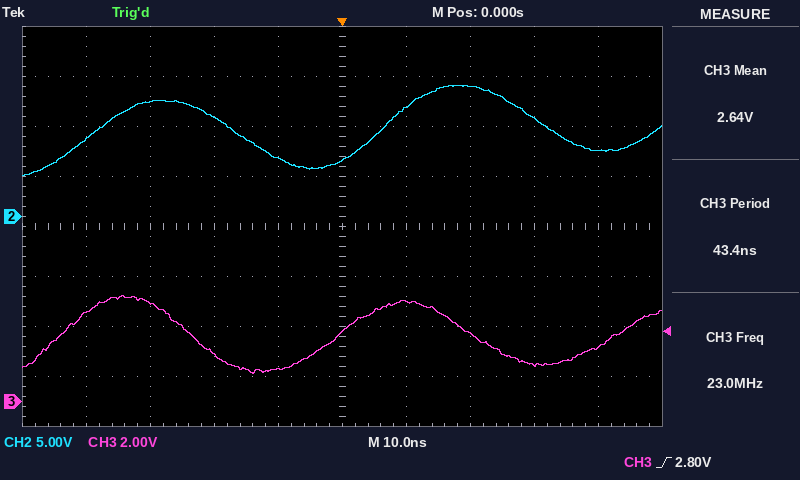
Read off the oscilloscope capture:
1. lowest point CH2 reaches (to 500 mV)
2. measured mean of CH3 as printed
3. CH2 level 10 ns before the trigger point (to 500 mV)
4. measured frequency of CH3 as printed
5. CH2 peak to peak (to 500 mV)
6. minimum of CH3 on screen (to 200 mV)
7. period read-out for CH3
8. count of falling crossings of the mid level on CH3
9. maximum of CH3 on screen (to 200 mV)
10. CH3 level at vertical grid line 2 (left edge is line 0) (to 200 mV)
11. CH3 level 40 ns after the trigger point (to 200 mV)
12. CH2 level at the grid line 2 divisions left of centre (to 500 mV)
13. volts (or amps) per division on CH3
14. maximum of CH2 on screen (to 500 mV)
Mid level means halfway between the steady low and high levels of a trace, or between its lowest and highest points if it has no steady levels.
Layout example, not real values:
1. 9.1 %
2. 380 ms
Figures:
1. 4.0 V
2. 2.64 V
3. 6.0 V
4. 23.0 MHz
5. 9.0 V
6. 1.2 V
7. 43.4 ns
8. 2
9. 4.2 V
10. 4.0 V
11. 2.2 V
12. 10.0 V
13. 2 V
14. 13.0 V
